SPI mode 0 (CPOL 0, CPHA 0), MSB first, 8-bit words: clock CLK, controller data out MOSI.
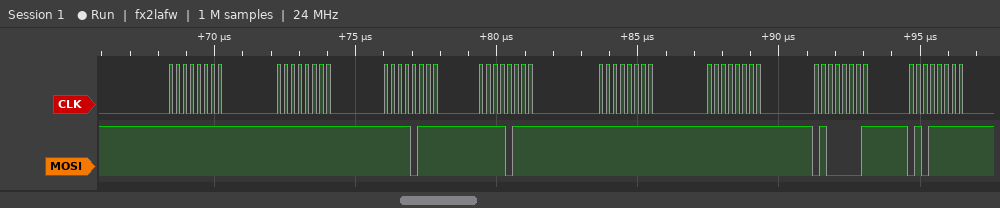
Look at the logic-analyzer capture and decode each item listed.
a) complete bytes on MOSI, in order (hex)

FF FF F7 F7 FF FF 41 5F
